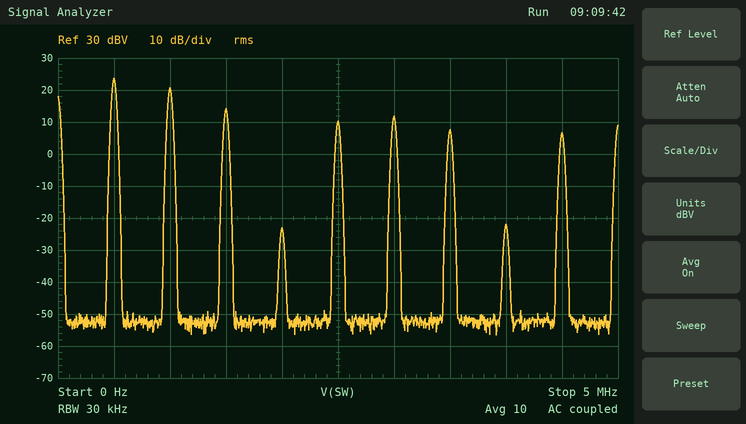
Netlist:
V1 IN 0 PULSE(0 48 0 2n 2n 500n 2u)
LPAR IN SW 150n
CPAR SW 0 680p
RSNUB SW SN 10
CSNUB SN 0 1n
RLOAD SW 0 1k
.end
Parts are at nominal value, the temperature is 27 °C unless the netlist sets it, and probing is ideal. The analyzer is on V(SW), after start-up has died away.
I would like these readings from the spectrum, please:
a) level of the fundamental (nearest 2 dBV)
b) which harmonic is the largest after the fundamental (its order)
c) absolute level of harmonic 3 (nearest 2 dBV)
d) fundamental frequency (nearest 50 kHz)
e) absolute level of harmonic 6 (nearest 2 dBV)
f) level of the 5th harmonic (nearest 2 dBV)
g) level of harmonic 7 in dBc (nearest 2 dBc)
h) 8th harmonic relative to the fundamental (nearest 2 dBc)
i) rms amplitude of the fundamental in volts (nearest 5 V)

24 dBV
2
14 dBV
500 kHz
12 dBV
10 dBV
-16 dBc
-46 dBc
15 V
